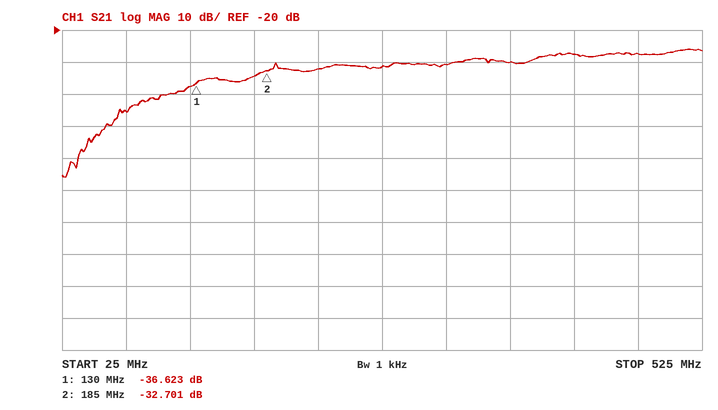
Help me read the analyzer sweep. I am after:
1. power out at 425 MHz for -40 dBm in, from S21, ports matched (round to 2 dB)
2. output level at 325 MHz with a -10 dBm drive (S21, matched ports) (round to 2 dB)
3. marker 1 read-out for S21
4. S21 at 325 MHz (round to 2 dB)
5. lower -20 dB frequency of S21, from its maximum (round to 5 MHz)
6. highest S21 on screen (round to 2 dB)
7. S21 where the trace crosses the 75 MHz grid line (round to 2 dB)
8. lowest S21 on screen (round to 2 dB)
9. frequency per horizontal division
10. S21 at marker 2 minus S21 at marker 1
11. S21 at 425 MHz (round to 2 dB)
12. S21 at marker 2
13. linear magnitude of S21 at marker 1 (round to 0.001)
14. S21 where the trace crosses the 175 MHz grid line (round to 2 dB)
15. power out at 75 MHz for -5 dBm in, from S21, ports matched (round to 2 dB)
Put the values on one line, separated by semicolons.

-68 dBm; -40 dBm; -36.623 dB; -30 dB; 70 MHz; -26 dB; -46 dB; -66 dB; 50 MHz; 3.922 dB; -28 dB; -32.701 dB; 0.015; -34 dB; -50 dBm
